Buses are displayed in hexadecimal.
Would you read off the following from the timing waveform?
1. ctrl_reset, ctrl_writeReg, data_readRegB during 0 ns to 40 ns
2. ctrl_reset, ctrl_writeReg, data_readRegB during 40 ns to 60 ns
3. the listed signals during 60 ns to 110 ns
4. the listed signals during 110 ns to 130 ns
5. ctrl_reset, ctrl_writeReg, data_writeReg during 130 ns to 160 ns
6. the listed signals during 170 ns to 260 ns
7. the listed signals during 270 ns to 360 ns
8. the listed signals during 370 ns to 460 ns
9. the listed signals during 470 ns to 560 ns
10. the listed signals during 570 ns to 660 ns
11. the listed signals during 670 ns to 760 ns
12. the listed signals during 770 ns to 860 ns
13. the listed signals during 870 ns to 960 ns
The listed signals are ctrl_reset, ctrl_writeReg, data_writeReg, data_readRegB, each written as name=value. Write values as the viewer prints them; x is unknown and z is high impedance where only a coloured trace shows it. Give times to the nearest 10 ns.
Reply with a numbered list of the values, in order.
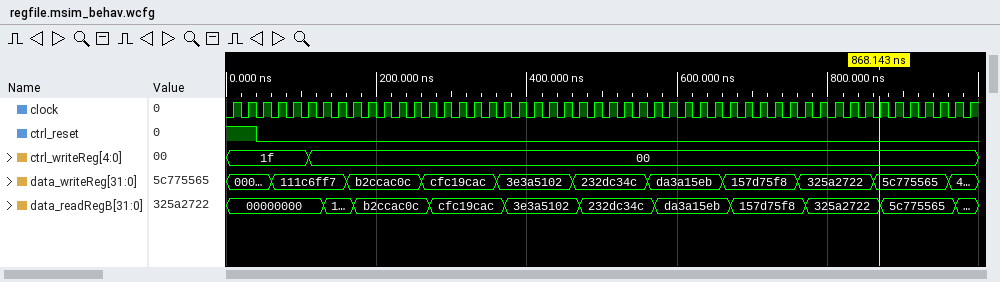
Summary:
1. ctrl_reset=1, ctrl_writeReg=1f, data_readRegB=00000000
2. ctrl_reset=0, ctrl_writeReg=1f, data_readRegB=00000000
3. ctrl_reset=0, ctrl_writeReg=1f, data_writeReg=111c6ff7, data_readRegB=00000000
4. ctrl_reset=0, ctrl_writeReg=00, data_writeReg=111c6ff7, data_readRegB=00000000
5. ctrl_reset=0, ctrl_writeReg=00, data_writeReg=111c6ff7
6. ctrl_reset=0, ctrl_writeReg=00, data_writeReg=b2ccac0c, data_readRegB=b2ccac0c
7. ctrl_reset=0, ctrl_writeReg=00, data_writeReg=cfc19cac, data_readRegB=cfc19cac
8. ctrl_reset=0, ctrl_writeReg=00, data_writeReg=3e3a5102, data_readRegB=3e3a5102
9. ctrl_reset=0, ctrl_writeReg=00, data_writeReg=232dc34c, data_readRegB=232dc34c
10. ctrl_reset=0, ctrl_writeReg=00, data_writeReg=da3a15eb, data_readRegB=da3a15eb
11. ctrl_reset=0, ctrl_writeReg=00, data_writeReg=157d75f8, data_readRegB=157d75f8
12. ctrl_reset=0, ctrl_writeReg=00, data_writeReg=325a2722, data_readRegB=325a2722
13. ctrl_reset=0, ctrl_writeReg=00, data_writeReg=5c775565, data_readRegB=5c775565
